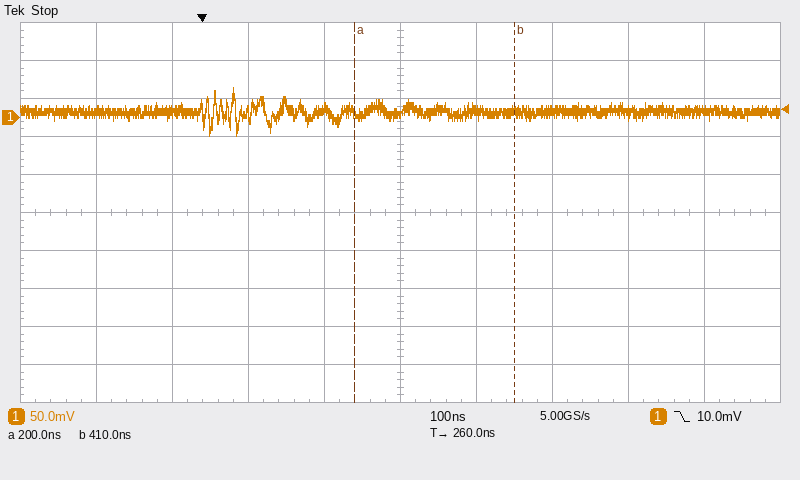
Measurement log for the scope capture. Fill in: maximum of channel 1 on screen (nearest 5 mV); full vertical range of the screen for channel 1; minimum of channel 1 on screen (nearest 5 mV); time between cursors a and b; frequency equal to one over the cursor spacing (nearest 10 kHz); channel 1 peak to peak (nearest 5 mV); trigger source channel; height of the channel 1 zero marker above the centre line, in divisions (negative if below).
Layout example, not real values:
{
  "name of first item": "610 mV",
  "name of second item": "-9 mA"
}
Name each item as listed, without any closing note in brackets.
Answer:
{
  "maximum of channel 1 on screen": "40 mV",
  "full vertical range of the screen for channel 1": "500 mV",
  "minimum of channel 1 on screen": "-25 mV",
  "time between cursors a and b": "210 ns",
  "frequency equal to one over the cursor spacing": "4.76 MHz",
  "channel 1 peak to peak": "65 mV",
  "trigger source channel": "channel 1",
  "height of the channel 1 zero marker above the centre line, in divisions": "+2.5 div"
}
